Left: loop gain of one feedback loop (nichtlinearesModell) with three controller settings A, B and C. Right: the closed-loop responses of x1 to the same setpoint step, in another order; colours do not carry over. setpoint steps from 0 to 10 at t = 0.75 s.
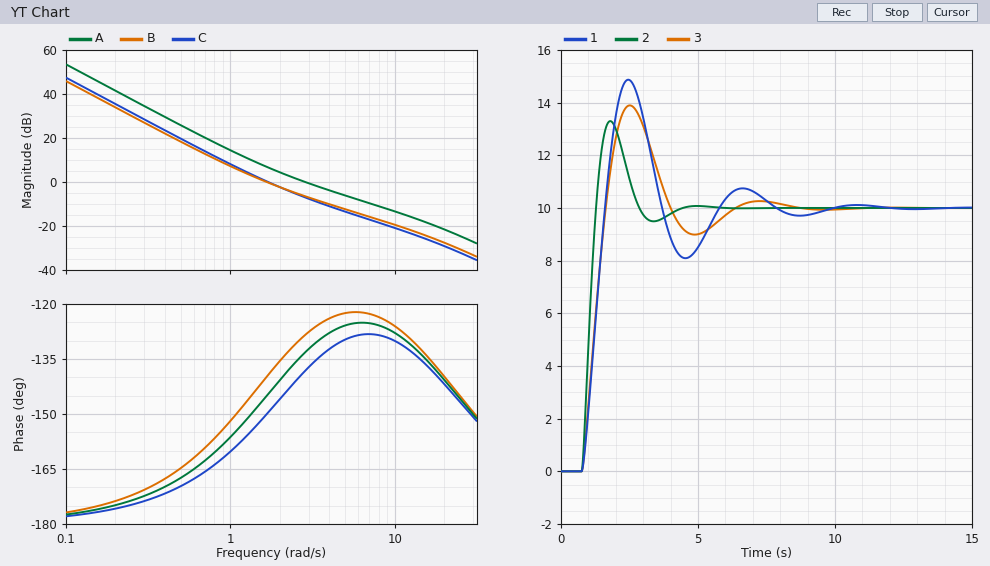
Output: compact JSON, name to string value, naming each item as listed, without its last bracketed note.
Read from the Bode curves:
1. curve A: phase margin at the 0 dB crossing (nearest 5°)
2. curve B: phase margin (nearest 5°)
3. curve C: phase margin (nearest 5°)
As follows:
{"curve A: phase margin at the 0 dB crossing": "45°", "curve B: phase margin": "40°", "curve C: phase margin": "30°"}
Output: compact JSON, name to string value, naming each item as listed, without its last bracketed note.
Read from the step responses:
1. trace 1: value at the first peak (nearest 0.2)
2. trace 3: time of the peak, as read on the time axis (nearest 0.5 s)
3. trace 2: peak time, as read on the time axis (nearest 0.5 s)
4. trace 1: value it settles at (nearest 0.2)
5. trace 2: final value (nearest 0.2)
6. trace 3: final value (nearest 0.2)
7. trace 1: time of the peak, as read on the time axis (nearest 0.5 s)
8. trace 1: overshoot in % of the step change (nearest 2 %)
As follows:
{"trace 1: value at the first peak": "14.8", "trace 3: time of the peak, as read on the time axis": "2.5 s", "trace 2: peak time, as read on the time axis": "2.0 s", "trace 1: value it settles at": "10.0", "trace 2: final value": "10.0", "trace 3: final value": "10.0", "trace 1: time of the peak, as read on the time axis": "2.5 s", "trace 1: overshoot in % of the step change": "48 %"}
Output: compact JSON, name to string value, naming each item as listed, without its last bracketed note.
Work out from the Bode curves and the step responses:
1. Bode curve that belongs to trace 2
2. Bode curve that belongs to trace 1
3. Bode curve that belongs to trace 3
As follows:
{"Bode curve that belongs to trace 2": "A", "Bode curve that belongs to trace 1": "C", "Bode curve that belongs to trace 3": "B"}
